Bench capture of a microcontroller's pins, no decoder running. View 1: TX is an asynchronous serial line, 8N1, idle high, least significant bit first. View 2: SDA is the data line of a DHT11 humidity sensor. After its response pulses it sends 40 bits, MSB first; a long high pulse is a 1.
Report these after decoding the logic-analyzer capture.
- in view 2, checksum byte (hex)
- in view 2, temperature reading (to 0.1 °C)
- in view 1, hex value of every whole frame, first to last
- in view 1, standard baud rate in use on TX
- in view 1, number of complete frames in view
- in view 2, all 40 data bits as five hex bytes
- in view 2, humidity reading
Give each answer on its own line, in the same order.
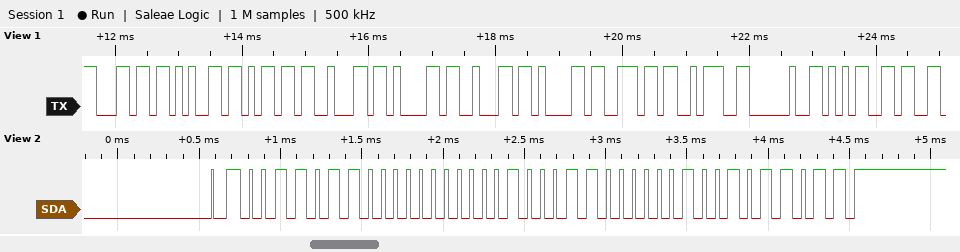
0x5B
35.2 °C
6C 65 6D 62 61 62 61 6E 3A 20 35
9600 baud
11
36 00 23 02 5B
54 %
